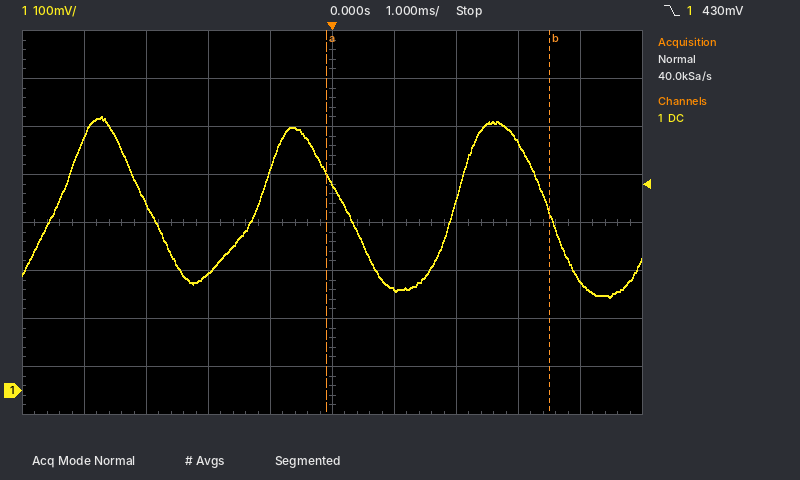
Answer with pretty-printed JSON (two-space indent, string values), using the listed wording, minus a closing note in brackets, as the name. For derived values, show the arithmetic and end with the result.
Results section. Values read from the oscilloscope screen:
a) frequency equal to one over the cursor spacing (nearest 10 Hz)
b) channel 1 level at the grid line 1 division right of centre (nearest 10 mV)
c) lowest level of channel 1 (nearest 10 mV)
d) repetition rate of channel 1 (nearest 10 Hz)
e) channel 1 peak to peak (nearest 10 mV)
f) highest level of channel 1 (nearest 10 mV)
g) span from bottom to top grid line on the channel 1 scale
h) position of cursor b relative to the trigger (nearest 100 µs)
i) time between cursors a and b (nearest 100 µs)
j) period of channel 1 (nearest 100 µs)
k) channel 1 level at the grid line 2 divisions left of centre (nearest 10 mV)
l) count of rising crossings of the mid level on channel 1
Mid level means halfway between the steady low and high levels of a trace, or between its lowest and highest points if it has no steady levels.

{
  "frequency equal to one over the cursor spacing": "1 / 3.6 ms ≈ 280 Hz",
  "channel 1 level at the grid line 1 division right of centre": "210 mV",
  "lowest level of channel 1": "190 mV",
  "repetition rate of channel 1": "1 / 3.2 ms ≈ 312 Hz, so 310 Hz to the nearest 10 Hz",
  "channel 1 peak to peak": "570 mV − (190 mV) = 380 mV",
  "highest level of channel 1": "570 mV",
  "span from bottom to top grid line on the channel 1 scale": "800 mV",
  "position of cursor b relative to the trigger": "+3.5 ms",
  "time between cursors a and b": "3.6 ms",
  "period of channel 1": "3.2 ms",
  "channel 1 level at the grid line 2 divisions left of centre": "240 mV",
  "count of rising crossings of the mid level on channel 1": "3"
}
